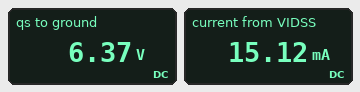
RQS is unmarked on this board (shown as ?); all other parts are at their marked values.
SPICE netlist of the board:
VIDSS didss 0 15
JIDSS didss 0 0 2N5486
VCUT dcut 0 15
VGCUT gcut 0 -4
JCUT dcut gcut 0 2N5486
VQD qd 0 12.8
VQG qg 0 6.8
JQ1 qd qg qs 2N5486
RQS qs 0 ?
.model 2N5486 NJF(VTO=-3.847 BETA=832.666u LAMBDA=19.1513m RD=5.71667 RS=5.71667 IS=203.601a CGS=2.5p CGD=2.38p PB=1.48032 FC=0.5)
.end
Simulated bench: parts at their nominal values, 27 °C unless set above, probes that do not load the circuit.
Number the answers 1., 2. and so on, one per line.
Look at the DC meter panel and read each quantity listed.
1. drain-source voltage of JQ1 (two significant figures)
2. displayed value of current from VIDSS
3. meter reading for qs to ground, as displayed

1. 6.4 V
2. 15.12 mA
3. 6.37 V
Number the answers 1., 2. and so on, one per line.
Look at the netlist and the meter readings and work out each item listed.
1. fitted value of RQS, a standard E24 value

1. 390 Ω
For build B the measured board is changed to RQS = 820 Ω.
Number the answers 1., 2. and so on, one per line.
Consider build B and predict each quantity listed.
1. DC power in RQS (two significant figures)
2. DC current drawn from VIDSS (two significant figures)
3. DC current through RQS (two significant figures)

1. 68 mW
2. 15 mA
3. 9.1 mA
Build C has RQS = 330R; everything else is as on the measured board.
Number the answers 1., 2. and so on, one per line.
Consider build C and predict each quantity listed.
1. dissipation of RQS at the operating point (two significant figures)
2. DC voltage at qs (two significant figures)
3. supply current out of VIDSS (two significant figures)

1. 110 mW
2. 6.1 V
3. 15 mA
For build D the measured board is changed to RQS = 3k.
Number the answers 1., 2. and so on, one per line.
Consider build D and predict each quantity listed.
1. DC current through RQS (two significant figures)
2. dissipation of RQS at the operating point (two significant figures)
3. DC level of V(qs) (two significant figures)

1. 2.9 mA
2. 26 mW
3. 8.8 V
